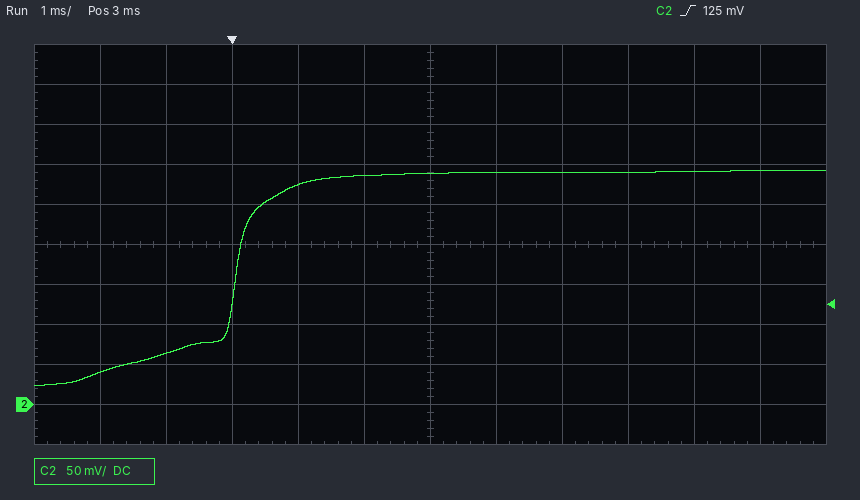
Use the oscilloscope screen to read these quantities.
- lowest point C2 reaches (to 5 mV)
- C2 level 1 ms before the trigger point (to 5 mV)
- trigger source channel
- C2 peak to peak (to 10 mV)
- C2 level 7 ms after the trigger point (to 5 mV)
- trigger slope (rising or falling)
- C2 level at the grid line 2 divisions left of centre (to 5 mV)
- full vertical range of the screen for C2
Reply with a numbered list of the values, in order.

1. 25 mV
2. 65 mV
3. C2
4. 270 mV
5. 290 mV
6. rising
7. 275 mV
8. 500 mV
